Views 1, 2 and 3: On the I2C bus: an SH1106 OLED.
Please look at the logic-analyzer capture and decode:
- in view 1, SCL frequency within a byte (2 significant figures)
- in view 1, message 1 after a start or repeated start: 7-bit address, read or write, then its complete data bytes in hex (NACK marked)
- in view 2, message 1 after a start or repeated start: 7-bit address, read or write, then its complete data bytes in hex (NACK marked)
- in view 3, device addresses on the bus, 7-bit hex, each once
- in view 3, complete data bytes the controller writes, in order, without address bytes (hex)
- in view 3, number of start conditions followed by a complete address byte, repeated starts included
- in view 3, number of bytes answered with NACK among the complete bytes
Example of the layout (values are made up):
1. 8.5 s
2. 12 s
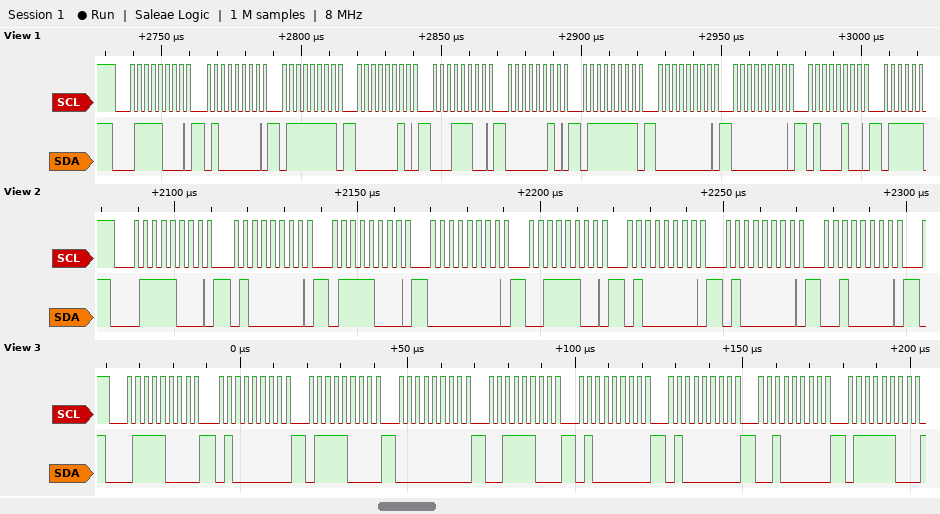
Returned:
1. 400 kHz
2. 0x3C write: 40 7F 02 1C 02 7F 00 00 44
3. 0x3C write: 40 78 00 3C 40 40 20
4. 0x3C
5. 40 78 00 3C 40 40 20 7C
6. 1
7. 0
